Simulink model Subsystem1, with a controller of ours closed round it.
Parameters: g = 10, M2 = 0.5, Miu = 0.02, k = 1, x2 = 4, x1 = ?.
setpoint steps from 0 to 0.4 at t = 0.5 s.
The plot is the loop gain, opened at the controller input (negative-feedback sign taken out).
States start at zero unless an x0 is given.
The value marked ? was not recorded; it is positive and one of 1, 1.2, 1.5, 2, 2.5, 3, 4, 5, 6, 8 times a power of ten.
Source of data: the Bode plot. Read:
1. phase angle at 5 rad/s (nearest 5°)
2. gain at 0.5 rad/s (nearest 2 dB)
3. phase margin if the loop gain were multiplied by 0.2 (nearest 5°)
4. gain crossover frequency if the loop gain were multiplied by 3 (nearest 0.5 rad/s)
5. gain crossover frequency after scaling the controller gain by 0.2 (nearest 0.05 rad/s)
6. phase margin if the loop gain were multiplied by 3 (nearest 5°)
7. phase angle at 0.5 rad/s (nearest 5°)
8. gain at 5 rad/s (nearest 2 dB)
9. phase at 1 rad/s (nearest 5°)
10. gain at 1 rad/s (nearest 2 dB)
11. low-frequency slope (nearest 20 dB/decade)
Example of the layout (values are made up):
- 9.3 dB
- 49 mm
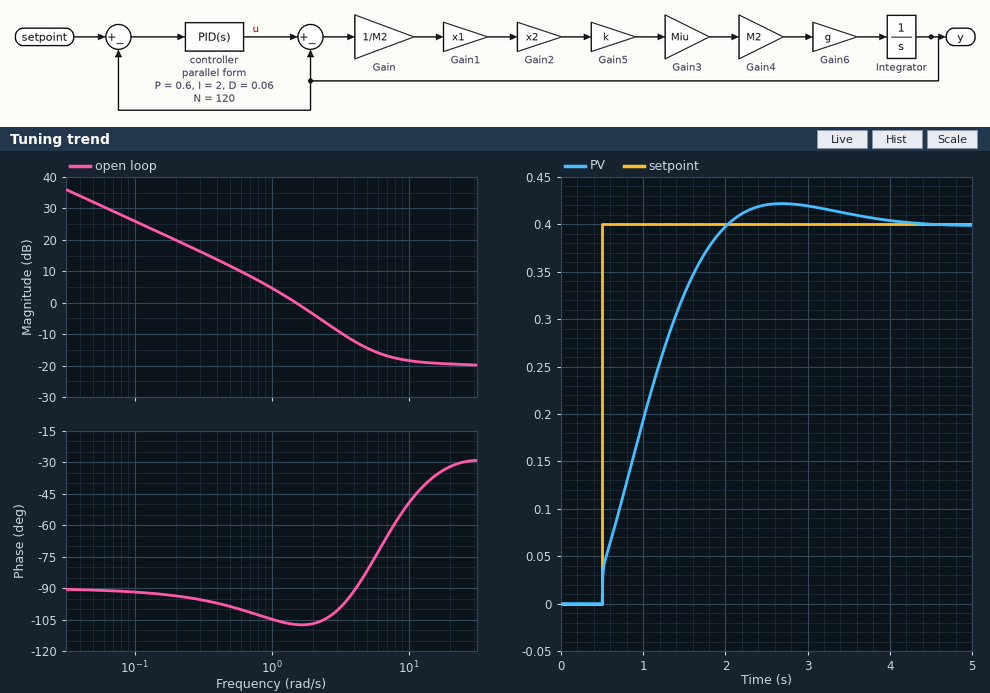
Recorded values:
- -80°
- 12 dB
- 85°
- 3.0 rad/s
- 0.40 rad/s
- 80°
- -100°
- -14 dB
- -105°
- 4 dB
- -20 dB/decade
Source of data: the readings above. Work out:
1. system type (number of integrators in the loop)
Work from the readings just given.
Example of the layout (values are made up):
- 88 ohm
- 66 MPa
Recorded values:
- 1
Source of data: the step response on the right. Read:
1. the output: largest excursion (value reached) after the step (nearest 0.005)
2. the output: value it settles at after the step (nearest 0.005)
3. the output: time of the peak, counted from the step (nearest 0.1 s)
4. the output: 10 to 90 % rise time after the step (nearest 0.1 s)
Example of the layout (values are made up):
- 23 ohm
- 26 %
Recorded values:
- 0.420
- 0.400
- 2.2 s
- 1.2 s
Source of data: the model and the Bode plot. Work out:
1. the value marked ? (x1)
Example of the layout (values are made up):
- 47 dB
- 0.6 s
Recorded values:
- 2
